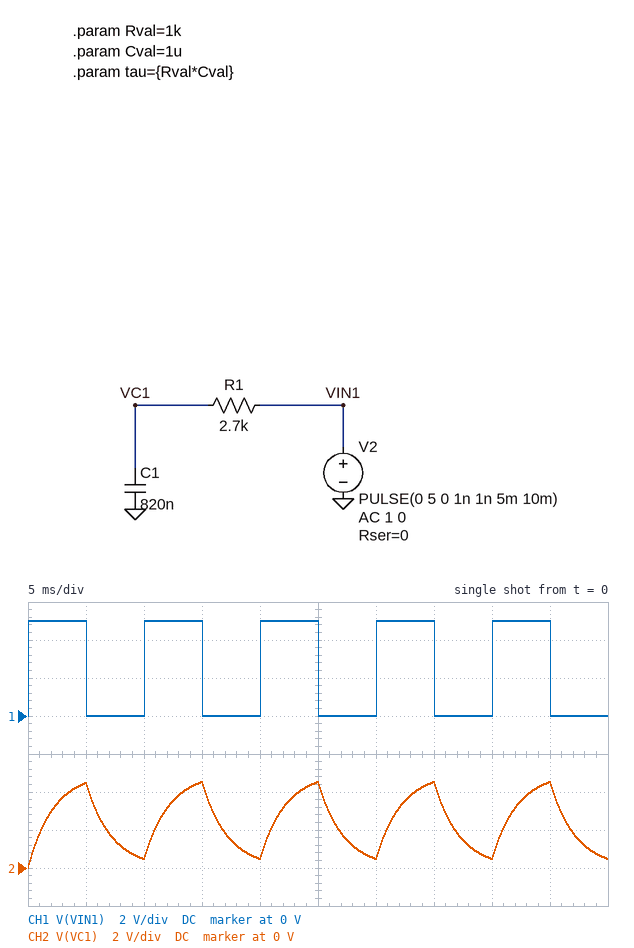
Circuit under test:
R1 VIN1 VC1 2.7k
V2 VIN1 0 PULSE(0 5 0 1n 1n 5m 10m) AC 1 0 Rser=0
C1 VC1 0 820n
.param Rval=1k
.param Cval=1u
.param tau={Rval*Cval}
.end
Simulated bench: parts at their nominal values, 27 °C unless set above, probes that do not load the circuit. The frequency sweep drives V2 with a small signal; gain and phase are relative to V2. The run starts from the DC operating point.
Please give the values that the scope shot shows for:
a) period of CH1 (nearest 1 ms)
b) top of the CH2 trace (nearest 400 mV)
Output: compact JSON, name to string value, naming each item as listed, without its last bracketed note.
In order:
{"period of CH1": "10 ms", "top of the CH2 trace": "4.4 V"}
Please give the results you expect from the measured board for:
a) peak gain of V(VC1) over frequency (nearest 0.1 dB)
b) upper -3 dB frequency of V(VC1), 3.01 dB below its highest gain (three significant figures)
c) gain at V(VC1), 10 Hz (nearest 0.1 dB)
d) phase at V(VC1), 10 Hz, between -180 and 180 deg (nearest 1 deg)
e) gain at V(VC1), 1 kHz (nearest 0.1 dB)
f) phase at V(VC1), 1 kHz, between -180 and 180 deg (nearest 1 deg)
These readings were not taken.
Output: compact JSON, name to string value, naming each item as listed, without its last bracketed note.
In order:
{"peak gain of V(VC1) over frequency": "0 dB", "upper -3 dB frequency of V(VC1), 3.01 dB below its highest gain": "71.9 Hz", "gain at V(VC1), 10 Hz": "-0.1 dB", "phase at V(VC1), 10 Hz, between -180 and 180 deg": "-8 deg", "gain at V(VC1), 1 kHz": "-22.9 dB", "phase at V(VC1), 1 kHz, between -180 and 180 deg": "-86 deg"}
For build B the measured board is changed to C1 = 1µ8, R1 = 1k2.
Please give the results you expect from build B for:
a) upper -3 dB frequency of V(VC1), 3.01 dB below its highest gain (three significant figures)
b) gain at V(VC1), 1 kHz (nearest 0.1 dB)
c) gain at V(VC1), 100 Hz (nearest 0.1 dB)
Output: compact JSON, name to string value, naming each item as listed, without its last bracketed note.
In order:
{"upper -3 dB frequency of V(VC1), 3.01 dB below its highest gain": "73.7 Hz", "gain at V(VC1), 1 kHz": "-22.7 dB", "gain at V(VC1), 100 Hz": "-4.5 dB"}
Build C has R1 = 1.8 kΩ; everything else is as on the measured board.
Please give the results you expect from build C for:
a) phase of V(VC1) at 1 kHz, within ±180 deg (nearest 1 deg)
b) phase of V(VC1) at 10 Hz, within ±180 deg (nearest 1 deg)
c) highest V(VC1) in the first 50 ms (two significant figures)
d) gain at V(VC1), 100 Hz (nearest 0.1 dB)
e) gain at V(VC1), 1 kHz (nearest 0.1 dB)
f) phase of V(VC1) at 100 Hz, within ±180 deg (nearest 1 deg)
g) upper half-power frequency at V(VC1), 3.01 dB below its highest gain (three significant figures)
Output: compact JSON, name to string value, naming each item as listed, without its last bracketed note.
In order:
{"phase of V(VC1) at 1 kHz, within ±180 deg": "-84 deg", "phase of V(VC1) at 10 Hz, within ±180 deg": "-5 deg", "highest V(VC1) in the first 50 ms": "4.8 V", "gain at V(VC1), 100 Hz": "-2.7 dB", "gain at V(VC1), 1 kHz": "-19.4 dB", "phase of V(VC1) at 100 Hz, within ±180 deg": "-43 deg", "upper half-power frequency at V(VC1), 3.01 dB below its highest gain": "108 Hz"}
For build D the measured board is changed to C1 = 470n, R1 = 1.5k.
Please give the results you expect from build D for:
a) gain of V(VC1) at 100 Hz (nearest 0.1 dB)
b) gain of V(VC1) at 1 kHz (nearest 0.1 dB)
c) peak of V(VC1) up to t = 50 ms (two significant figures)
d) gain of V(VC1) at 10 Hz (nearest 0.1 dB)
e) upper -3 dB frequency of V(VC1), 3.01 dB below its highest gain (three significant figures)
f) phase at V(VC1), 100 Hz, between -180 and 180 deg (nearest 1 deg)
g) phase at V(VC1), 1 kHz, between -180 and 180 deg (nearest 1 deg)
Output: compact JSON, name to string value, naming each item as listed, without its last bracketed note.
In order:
{"gain of V(VC1) at 100 Hz": "-0.8 dB", "gain of V(VC1) at 1 kHz": "-13.1 dB", "peak of V(VC1) up to t = 50 ms": "5.0 V", "gain of V(VC1) at 10 Hz": "0 dB", "upper -3 dB frequency of V(VC1), 3.01 dB below its highest gain": "226 Hz", "phase at V(VC1), 100 Hz, between -180 and 180 deg": "-24 deg", "phase at V(VC1), 1 kHz, between -180 and 180 deg": "-77 deg"}
